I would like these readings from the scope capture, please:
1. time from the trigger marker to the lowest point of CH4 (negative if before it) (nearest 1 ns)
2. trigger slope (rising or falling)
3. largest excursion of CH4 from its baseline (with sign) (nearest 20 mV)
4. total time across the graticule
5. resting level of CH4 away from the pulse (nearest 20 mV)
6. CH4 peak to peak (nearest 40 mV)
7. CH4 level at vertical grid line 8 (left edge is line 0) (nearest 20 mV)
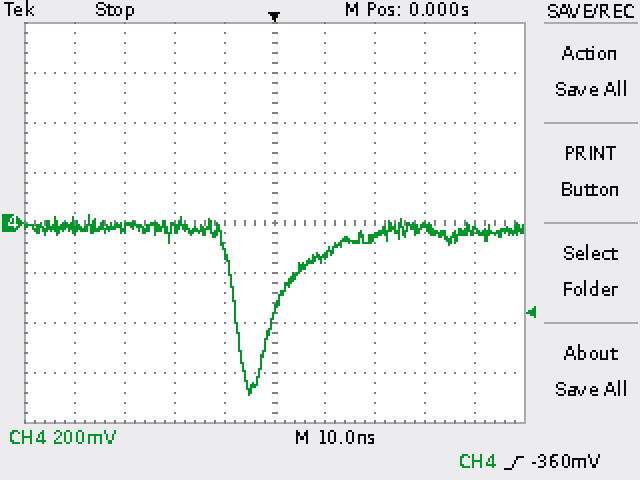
-5 ns
rising
-660 mV
100 ns
-20 mV
720 mV
-20 mV
